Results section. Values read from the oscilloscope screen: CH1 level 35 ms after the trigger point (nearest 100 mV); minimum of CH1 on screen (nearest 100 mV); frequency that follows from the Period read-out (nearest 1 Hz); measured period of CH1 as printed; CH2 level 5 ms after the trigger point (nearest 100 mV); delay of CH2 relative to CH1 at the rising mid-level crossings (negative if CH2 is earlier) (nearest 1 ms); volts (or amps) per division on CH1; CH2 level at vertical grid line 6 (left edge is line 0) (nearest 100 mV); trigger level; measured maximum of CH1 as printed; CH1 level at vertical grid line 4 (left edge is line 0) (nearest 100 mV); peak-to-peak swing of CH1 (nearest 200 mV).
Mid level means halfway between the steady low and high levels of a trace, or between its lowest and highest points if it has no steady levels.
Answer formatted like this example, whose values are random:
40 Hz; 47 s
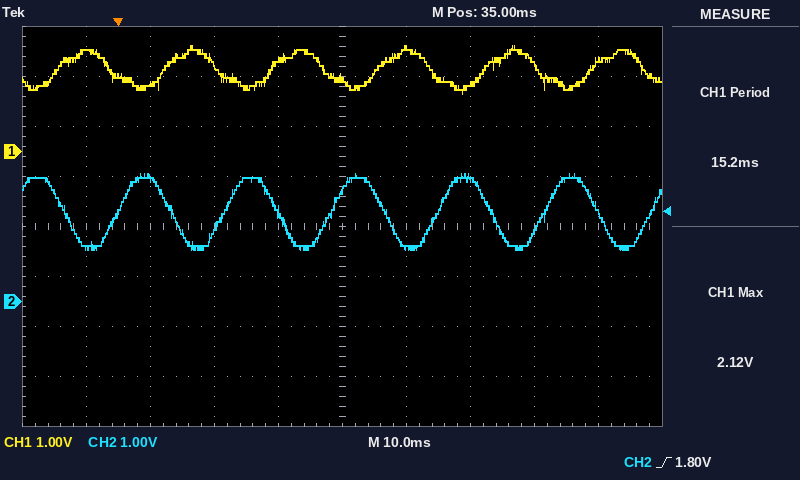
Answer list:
1.5 V; 1.2 V; 66 Hz; 15.2 ms; 2.5 V; -7 ms; 1 V; 1.1 V; 1.80 V; 2.12 V; 1.8 V; 1.0 V
